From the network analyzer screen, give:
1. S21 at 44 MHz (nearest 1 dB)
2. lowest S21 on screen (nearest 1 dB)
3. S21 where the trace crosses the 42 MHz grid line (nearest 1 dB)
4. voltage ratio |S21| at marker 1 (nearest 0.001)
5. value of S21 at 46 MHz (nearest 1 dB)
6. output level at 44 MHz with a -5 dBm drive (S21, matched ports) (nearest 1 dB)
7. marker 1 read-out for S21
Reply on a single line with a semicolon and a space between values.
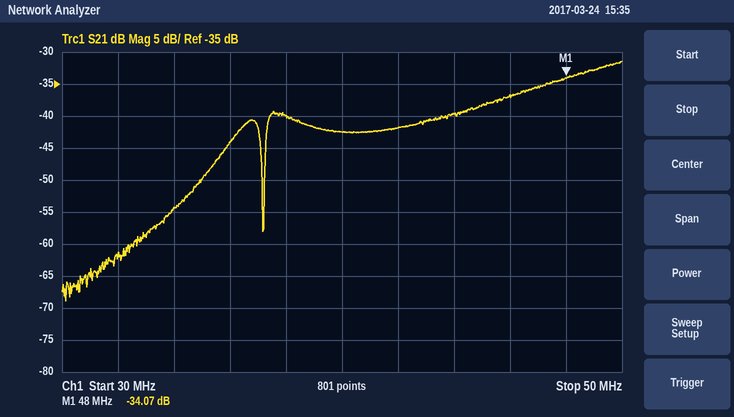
-40 dB; -69 dB; -42 dB; 0.020; -37 dB; -45 dBm; -34.07 dB
